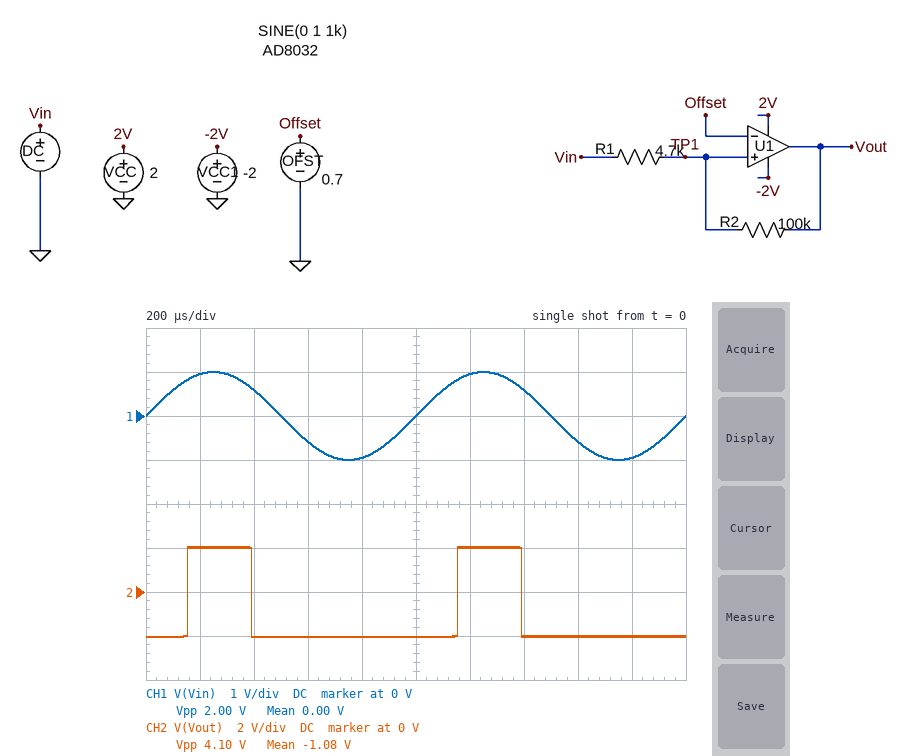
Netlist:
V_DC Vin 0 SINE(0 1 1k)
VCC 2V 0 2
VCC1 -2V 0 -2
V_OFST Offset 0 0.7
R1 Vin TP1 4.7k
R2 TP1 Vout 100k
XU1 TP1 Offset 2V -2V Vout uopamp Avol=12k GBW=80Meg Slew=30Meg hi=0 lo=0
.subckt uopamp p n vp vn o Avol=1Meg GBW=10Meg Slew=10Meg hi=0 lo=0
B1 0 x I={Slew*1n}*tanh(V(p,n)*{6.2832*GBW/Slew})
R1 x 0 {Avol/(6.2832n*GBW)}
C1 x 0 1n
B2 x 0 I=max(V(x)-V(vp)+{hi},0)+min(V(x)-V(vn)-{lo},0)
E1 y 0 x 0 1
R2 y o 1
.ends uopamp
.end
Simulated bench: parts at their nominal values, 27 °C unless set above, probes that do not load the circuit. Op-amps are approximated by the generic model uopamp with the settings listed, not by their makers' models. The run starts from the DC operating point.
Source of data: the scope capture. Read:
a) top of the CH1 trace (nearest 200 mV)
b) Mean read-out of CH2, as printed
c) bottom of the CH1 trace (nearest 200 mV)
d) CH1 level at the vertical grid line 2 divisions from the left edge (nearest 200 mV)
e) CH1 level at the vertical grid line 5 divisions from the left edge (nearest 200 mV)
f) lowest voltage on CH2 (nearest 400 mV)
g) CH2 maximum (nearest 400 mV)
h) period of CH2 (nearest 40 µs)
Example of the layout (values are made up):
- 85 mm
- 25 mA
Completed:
- 1.0 V
- -1.08 V
- -1.0 V
- 600 mV
- 0 V
- -2.0 V
- 2.0 V
- 1.00 ms
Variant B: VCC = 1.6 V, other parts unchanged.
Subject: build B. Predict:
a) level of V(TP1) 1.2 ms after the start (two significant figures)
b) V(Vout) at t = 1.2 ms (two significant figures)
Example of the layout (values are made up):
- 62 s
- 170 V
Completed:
- 980 mV
- 1.6 V
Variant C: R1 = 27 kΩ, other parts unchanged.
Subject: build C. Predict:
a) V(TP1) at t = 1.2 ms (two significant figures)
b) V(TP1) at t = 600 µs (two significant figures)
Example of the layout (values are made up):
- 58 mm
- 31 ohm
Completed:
- 320 mV
- -890 mV
